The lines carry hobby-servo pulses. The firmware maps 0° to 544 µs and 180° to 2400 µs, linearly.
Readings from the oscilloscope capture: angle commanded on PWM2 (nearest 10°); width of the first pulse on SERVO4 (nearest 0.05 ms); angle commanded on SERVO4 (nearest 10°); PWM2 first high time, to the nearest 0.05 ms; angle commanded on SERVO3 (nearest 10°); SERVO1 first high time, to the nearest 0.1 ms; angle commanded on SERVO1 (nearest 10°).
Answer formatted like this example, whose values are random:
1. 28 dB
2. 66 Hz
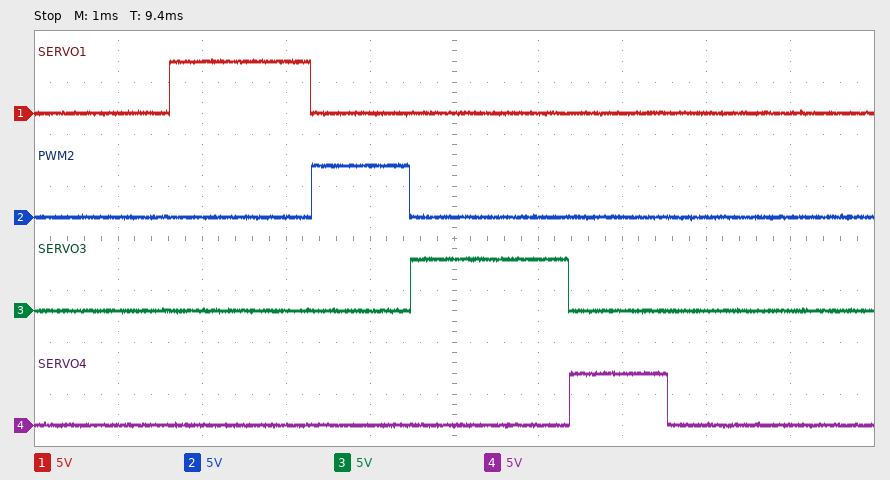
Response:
1. 60°
2. 1.15 ms
3. 60°
4. 1.15 ms
5. 130°
6. 1.7 ms
7. 110°
